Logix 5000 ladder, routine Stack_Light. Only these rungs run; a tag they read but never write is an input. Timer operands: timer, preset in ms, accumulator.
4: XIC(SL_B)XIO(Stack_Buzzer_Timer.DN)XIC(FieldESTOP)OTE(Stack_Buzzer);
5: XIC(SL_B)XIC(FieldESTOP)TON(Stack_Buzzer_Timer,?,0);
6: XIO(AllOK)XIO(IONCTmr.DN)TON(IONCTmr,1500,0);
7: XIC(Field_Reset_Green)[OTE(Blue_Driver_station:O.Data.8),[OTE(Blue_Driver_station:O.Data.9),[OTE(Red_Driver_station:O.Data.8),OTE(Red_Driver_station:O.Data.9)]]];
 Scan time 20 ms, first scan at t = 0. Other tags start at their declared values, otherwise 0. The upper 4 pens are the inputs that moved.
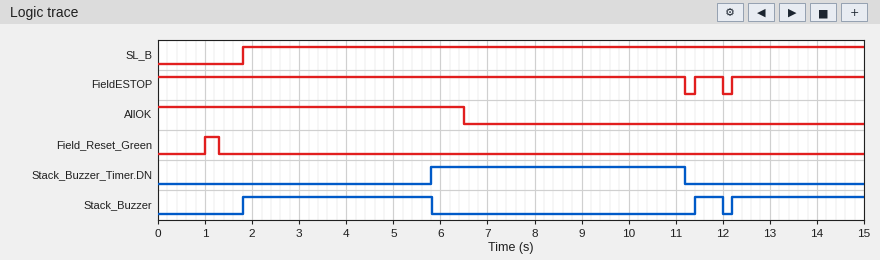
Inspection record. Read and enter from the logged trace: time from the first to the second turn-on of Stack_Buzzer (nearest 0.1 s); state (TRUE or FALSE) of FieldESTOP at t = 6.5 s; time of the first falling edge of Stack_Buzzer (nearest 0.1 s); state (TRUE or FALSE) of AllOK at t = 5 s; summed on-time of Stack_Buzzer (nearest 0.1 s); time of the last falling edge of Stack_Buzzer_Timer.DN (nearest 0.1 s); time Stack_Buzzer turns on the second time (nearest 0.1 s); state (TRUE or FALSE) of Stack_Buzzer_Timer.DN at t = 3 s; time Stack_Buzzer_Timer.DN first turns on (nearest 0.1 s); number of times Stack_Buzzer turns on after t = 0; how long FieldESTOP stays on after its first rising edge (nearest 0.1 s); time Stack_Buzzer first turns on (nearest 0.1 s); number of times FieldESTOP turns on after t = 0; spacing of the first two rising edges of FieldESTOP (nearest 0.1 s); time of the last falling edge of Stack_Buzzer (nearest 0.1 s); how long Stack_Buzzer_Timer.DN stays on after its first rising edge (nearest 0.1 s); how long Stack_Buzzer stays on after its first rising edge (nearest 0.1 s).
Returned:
9.6 s
TRUE
5.8 s
TRUE
7.4 s
11.2 s
11.4 s
FALSE
5.8 s
3
0.6 s
1.8 s
2
0.8 s
12.0 s
5.4 s
4.0 s
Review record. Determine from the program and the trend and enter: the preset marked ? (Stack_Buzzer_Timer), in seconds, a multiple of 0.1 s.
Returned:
4.0 s
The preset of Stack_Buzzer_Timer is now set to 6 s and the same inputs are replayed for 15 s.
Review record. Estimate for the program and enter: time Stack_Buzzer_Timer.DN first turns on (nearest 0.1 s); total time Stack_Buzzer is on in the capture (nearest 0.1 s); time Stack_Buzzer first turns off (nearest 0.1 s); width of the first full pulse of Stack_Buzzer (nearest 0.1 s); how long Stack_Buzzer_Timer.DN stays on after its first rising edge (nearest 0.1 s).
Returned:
7.8 s
9.4 s
7.8 s
6.0 s
3.4 s
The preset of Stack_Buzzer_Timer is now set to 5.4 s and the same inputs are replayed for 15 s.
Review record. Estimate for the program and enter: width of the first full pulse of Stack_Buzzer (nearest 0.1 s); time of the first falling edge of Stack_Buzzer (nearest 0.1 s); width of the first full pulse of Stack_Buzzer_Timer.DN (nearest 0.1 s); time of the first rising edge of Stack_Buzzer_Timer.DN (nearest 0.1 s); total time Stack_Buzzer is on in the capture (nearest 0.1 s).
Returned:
5.4 s
7.2 s
4.0 s
7.2 s
8.8 s
